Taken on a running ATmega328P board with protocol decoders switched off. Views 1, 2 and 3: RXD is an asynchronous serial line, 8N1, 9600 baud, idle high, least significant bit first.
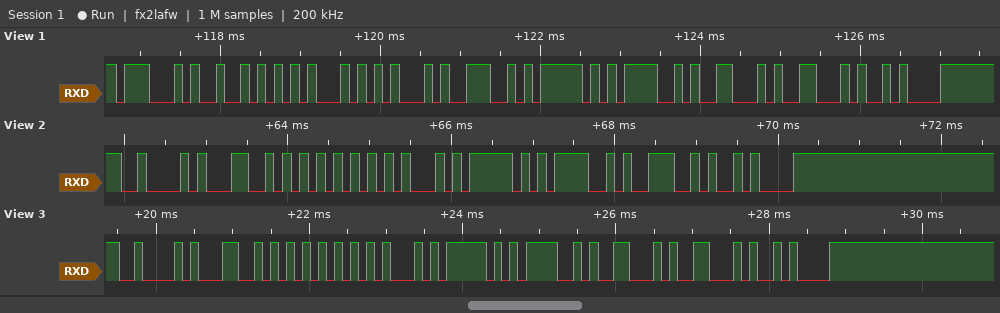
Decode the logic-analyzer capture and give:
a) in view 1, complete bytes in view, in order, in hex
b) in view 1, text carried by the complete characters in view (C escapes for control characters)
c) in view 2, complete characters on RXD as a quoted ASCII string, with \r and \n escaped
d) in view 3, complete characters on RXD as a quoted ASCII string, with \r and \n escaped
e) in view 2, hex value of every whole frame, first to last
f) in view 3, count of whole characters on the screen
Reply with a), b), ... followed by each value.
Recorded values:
a) 47 52 45 45 4E 5F 4F 46 46 0A
b) "GREEN_OFF\n"
c) "BLUE_ON\n"
d) "BLUE_OFF\n"
e) 0x42 0x4C 0x55 0x45 0x5F 0x4F 0x4E 0x0A
f) 9
